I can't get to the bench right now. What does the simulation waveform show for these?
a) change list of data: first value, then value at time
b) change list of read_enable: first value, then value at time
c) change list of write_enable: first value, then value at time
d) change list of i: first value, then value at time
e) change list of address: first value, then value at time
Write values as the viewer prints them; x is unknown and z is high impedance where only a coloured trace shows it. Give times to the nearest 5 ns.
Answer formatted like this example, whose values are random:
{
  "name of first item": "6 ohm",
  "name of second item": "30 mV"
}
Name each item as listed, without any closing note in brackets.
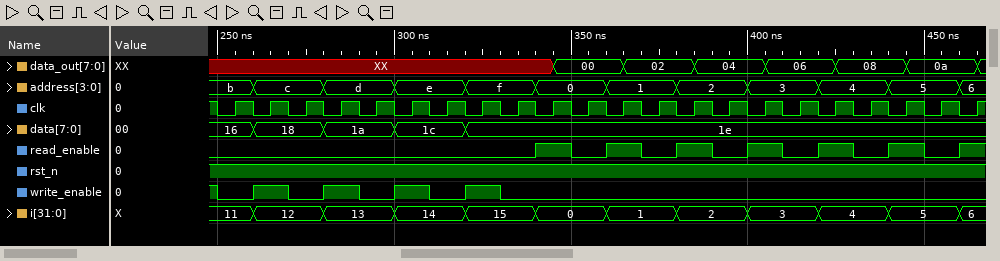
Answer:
{
  "change list of data: first value, then value at time": "16, 18 at 260 ns, 1a at 280 ns, 1c at 300 ns, 1e at 320 ns",
  "change list of read_enable: first value, then value at time": "0, 1 at 340 ns, 0 at 350 ns, 1 at 360 ns, 0 at 370 ns, 1 at 380 ns, 0 at 390 ns, 1 at 400 ns, 0 at 410 ns, 1 at 420 ns, 0 at 430 ns, 1 at 440 ns, 0 at 450 ns, 1 at 460 ns",
  "change list of write_enable: first value, then value at time": "1, 0 at 250 ns, 1 at 260 ns, 0 at 270 ns, 1 at 280 ns, 0 at 290 ns, 1 at 300 ns, 0 at 310 ns, 1 at 320 ns, 0 at 330 ns",
  "change list of i: first value, then value at time": "11, 12 at 260 ns, 13 at 280 ns, 14 at 300 ns, 15 at 320 ns, 0 at 340 ns, 1 at 360 ns, 2 at 380 ns, 3 at 400 ns, 4 at 420 ns, 5 at 440 ns, 6 at 460 ns",
  "change list of address: first value, then value at time": "b, c at 260 ns, d at 280 ns, e at 300 ns, f at 320 ns, 0 at 340 ns, 1 at 360 ns, 2 at 380 ns, 3 at 400 ns, 4 at 420 ns, 5 at 440 ns, 6 at 460 ns"
}
